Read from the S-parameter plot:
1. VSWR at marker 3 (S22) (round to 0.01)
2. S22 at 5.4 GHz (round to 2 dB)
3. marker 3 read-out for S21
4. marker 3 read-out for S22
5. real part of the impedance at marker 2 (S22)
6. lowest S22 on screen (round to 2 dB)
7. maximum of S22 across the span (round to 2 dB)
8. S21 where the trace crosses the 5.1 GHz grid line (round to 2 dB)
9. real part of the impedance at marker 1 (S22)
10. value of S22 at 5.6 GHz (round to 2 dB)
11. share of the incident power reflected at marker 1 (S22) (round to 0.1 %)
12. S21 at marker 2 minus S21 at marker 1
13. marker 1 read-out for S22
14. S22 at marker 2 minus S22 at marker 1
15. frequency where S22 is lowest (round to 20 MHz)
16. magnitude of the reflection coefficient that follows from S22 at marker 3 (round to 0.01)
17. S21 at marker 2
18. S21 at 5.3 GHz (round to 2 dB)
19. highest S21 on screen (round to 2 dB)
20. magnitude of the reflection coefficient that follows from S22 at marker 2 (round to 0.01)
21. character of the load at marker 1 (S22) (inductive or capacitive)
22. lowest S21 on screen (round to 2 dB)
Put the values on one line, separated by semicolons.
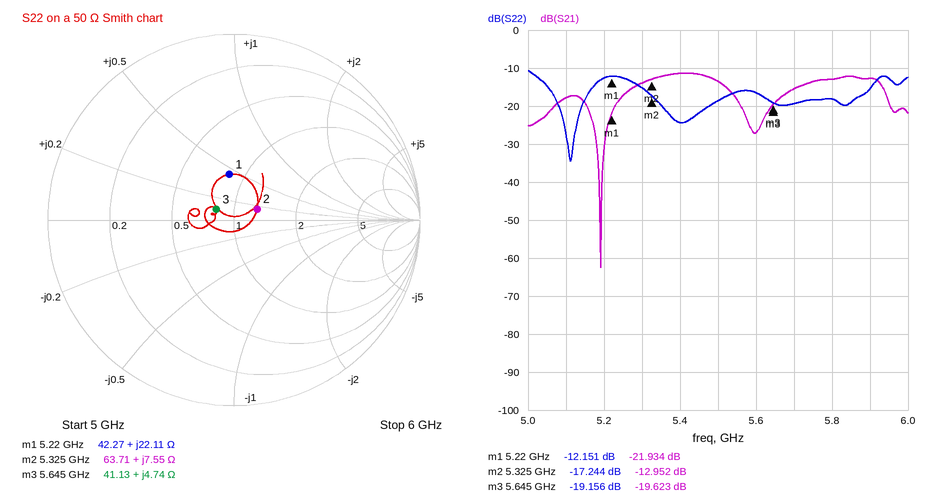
1.25; -24 dB; -19.623 dB; -19.156 dB; 63.71 Ω; -34 dB; -10 dB; -18 dB; 42.27 Ω; -16 dB; 6.1 %; 8.982 dB; -12.151 dB; -5.093 dB; 5.12 GHz; 0.11; -12.952 dB; -14 dB; -12 dB; 0.14; inductive; -62 dB
